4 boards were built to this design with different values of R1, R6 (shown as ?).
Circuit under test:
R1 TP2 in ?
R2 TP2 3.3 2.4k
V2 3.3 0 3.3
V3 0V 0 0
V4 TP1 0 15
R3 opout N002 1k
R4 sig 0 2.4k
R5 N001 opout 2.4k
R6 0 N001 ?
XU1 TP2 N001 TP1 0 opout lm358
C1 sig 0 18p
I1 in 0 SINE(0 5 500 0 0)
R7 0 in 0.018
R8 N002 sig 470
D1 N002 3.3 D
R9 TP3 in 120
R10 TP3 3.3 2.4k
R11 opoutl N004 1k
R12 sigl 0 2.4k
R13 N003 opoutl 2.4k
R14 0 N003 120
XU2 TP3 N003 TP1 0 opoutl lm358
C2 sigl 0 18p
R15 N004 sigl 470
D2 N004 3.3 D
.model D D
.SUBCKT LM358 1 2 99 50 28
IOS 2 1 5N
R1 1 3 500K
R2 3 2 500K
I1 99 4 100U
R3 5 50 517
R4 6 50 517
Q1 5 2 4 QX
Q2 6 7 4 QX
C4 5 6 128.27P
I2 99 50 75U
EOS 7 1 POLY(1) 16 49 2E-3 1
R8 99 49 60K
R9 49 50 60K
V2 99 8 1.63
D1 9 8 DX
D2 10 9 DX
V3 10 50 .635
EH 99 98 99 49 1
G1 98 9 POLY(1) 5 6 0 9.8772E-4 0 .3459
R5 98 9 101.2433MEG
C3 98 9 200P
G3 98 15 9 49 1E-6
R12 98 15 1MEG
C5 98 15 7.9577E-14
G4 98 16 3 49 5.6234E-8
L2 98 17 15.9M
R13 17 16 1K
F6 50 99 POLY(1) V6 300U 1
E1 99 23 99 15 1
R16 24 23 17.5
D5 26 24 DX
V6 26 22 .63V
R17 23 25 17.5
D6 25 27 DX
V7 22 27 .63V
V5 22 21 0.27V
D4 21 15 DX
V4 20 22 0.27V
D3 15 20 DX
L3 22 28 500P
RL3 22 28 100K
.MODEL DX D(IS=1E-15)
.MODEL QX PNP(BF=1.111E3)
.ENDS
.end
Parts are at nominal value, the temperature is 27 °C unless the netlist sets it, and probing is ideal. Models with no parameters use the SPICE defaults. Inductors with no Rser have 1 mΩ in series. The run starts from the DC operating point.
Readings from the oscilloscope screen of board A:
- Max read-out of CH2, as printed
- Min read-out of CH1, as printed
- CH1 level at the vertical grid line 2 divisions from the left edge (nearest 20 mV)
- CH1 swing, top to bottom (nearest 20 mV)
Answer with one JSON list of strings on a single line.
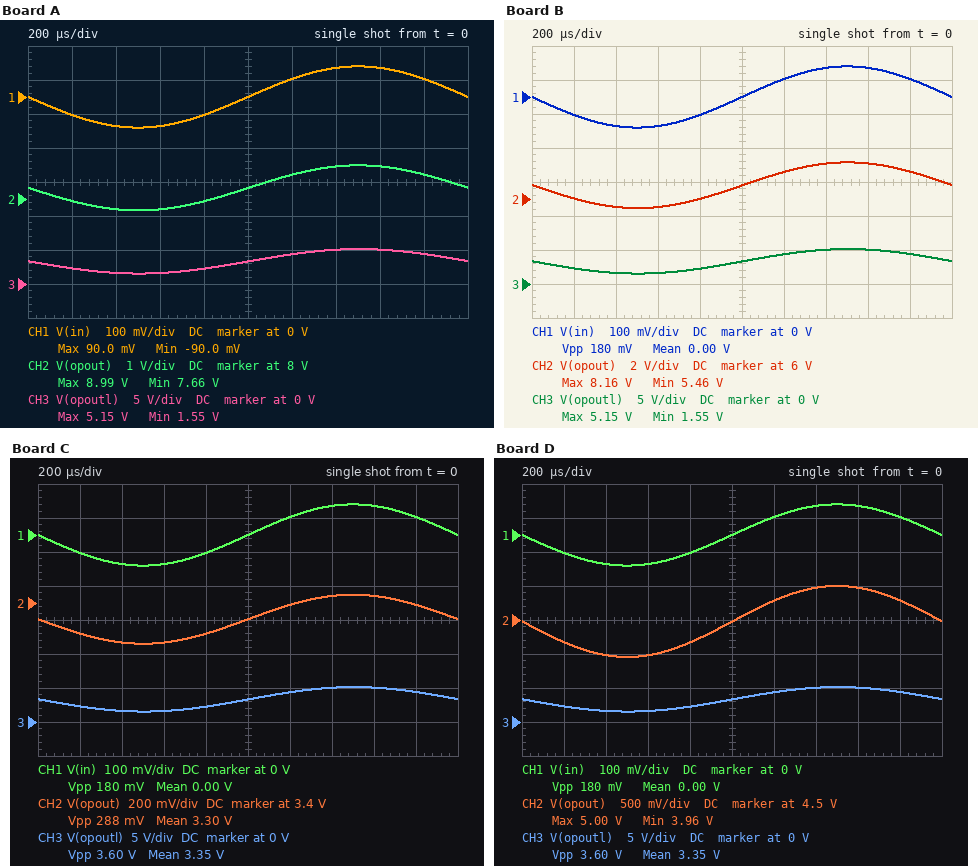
["8.99 V", "-90.0 mV", "-80 mV", "180 mV"]
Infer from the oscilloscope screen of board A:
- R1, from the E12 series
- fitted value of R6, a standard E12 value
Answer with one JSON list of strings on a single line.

["820 Ω", "270 Ω"]
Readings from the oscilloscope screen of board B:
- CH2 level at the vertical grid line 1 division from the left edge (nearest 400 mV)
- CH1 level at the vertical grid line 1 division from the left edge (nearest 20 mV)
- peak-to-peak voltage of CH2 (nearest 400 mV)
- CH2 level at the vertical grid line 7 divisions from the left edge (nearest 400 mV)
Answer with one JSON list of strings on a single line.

["6.0 V", "-60 mV", "2.8 V", "8.0 V"]
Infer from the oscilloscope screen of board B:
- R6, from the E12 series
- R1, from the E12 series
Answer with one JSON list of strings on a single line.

["150 Ω", "330 Ω"]
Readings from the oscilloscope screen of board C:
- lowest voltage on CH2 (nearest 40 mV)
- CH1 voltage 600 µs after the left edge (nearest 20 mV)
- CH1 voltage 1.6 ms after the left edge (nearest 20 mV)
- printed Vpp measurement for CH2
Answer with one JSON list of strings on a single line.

["3.16 V", "-80 mV", "80 mV", "288 mV"]
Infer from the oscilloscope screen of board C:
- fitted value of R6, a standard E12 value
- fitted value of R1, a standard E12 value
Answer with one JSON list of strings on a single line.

["1.5 kΩ", "1.5 kΩ"]
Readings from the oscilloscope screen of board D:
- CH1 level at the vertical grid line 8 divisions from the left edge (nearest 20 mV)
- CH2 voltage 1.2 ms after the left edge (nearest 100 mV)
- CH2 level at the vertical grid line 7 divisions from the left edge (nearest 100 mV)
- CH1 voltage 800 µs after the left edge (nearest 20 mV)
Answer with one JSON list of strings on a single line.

["80 mV", "4.8 V", "5.0 V", "-60 mV"]
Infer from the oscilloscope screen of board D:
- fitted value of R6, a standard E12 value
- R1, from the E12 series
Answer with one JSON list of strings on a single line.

["390 Ω", "560 Ω"]
